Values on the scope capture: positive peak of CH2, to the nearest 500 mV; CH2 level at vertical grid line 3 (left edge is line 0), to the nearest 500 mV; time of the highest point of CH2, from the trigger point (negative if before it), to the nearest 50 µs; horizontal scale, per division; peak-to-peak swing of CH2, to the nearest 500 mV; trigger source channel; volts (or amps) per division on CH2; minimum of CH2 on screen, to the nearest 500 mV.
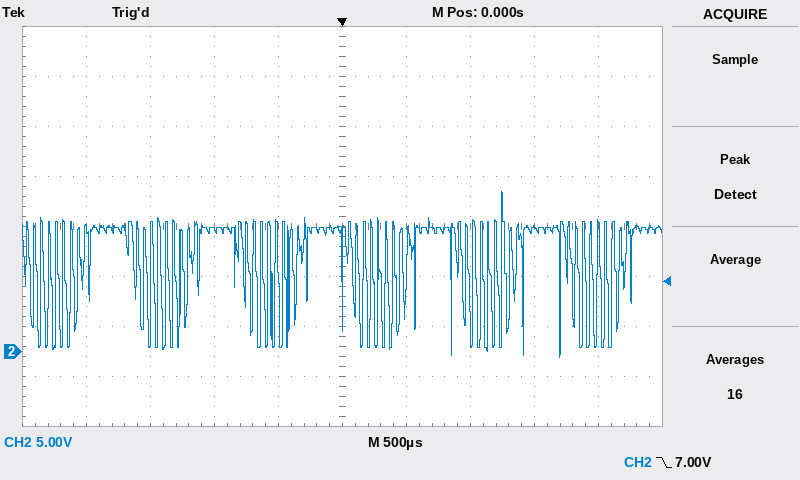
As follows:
16.0 V
12.0 V
+1.25 ms
500 µs
16.5 V
CH2
5 V
-500 mV
